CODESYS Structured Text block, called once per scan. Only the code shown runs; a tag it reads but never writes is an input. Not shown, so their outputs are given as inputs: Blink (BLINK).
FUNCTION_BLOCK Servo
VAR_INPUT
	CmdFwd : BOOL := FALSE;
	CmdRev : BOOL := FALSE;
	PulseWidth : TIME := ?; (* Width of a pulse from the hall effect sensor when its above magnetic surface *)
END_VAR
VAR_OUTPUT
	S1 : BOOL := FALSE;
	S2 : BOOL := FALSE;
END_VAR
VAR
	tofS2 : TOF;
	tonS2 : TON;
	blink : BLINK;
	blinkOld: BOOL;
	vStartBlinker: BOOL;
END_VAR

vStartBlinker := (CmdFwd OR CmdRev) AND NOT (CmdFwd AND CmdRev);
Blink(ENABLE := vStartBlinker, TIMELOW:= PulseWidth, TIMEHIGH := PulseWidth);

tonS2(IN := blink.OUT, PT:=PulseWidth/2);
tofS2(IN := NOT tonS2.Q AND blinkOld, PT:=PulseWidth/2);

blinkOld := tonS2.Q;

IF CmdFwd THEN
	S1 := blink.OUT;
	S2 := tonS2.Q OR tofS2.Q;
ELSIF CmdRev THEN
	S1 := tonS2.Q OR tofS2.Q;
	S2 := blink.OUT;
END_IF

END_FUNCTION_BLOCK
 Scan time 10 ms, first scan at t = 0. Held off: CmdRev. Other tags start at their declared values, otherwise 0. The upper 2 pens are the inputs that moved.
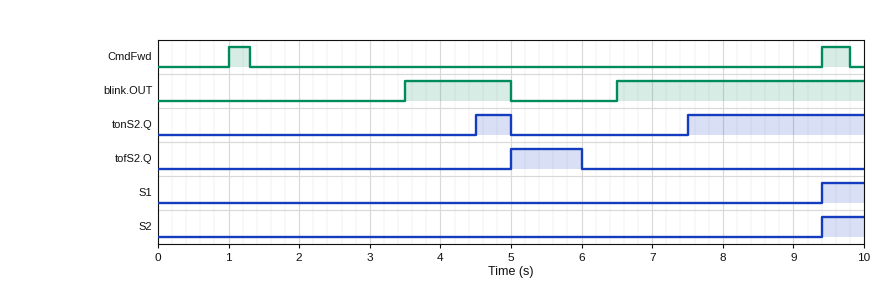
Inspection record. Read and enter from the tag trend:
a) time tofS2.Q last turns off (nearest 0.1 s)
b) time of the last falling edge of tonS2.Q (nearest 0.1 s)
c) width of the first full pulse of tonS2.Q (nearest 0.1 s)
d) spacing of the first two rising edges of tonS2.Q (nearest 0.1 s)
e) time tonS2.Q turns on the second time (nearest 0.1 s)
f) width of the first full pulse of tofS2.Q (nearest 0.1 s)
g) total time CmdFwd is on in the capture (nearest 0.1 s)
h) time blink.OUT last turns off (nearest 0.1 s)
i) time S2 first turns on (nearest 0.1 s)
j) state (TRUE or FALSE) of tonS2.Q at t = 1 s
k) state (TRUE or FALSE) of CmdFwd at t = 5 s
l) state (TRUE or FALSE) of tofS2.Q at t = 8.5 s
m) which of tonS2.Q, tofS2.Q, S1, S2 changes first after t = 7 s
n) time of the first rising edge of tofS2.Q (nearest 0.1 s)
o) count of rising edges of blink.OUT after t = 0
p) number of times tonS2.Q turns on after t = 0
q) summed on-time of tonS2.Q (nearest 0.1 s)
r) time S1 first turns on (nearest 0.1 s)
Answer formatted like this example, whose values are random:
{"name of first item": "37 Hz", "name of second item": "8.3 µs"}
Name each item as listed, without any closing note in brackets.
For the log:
{"time tofS2.Q last turns off": "6.0 s", "time of the last falling edge of tonS2.Q": "5.0 s", "width of the first full pulse of tonS2.Q": "0.5 s", "spacing of the first two rising edges of tonS2.Q": "3.0 s", "time tonS2.Q turns on the second time": "7.5 s", "width of the first full pulse of tofS2.Q": "1.0 s", "total time CmdFwd is on in the capture": "0.7 s", "time blink.OUT last turns off": "5.0 s", "time S2 first turns on": "9.4 s", "state (TRUE or FALSE) of tonS2.Q at t = 1 s": "FALSE", "state (TRUE or FALSE) of CmdFwd at t = 5 s": "FALSE", "state (TRUE or FALSE) of tofS2.Q at t = 8.5 s": "FALSE", "which of tonS2.Q, tofS2.Q, S1, S2 changes first after t = 7 s": "tonS2.Q", "time of the first rising edge of tofS2.Q": "5.0 s", "count of rising edges of blink.OUT after t = 0": "2", "number of times tonS2.Q turns on after t = 0": "2", "summed on-time of tonS2.Q": "3.0 s", "time S1 first turns on": "9.4 s"}
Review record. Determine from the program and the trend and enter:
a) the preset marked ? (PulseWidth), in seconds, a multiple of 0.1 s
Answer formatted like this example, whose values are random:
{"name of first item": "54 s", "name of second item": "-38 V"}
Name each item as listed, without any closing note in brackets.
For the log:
{"the preset marked ? (PulseWidth), in seconds, a multiple of 0.1 s": "2.0 s"}
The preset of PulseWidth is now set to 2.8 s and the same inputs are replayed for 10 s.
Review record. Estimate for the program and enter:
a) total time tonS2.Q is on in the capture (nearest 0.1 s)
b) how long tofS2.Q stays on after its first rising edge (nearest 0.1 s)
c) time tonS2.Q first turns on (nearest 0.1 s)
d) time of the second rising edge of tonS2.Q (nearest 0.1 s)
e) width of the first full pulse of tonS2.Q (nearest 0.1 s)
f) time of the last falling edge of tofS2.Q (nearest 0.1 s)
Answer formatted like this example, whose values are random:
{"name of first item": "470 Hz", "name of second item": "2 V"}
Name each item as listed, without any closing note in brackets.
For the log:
{"total time tonS2.Q is on in the capture": "2.2 s", "how long tofS2.Q stays on after its first rising edge": "1.4 s", "time tonS2.Q first turns on": "4.9 s", "time of the second rising edge of tonS2.Q": "7.9 s", "width of the first full pulse of tonS2.Q": "0.1 s", "time of the last falling edge of tofS2.Q": "6.4 s"}
